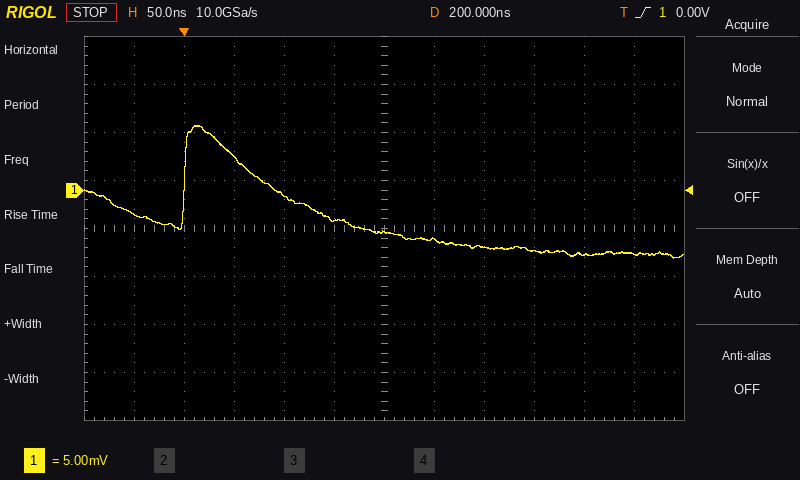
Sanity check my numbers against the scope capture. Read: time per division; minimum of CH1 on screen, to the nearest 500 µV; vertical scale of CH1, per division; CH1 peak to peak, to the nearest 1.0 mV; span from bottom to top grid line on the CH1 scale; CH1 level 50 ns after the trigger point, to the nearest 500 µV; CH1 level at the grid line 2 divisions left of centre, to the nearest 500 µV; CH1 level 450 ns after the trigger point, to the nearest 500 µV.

50 ns
-7.0 mV
5 mV
14.0 mV
40 mV
3.5 mV
-500 µV
-6.5 mV
